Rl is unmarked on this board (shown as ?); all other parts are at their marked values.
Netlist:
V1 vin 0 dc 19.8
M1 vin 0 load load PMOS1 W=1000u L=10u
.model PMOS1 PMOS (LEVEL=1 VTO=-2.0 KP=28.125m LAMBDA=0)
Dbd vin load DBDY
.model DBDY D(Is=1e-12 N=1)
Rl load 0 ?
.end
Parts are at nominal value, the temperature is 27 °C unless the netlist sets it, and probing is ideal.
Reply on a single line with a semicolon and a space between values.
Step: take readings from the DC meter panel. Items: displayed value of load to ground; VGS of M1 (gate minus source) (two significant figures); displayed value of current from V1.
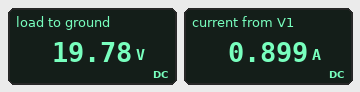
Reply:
19.78 V; -20 V; 0.899 A
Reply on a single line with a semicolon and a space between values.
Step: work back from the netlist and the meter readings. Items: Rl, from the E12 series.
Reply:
22 Ω
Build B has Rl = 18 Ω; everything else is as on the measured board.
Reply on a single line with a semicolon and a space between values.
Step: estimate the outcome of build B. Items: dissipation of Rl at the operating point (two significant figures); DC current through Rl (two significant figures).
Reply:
22 W; 1.1 A
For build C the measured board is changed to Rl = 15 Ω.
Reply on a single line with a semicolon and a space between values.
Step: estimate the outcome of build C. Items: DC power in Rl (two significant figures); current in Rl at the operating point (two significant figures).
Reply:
26 W; 1.3 A
